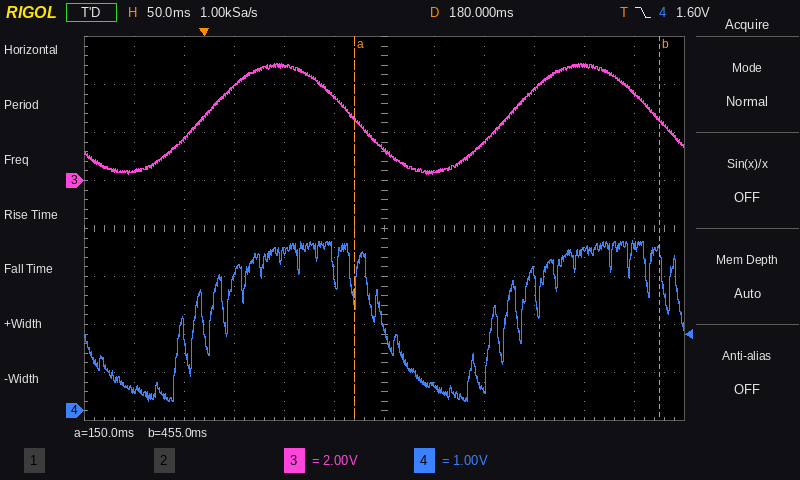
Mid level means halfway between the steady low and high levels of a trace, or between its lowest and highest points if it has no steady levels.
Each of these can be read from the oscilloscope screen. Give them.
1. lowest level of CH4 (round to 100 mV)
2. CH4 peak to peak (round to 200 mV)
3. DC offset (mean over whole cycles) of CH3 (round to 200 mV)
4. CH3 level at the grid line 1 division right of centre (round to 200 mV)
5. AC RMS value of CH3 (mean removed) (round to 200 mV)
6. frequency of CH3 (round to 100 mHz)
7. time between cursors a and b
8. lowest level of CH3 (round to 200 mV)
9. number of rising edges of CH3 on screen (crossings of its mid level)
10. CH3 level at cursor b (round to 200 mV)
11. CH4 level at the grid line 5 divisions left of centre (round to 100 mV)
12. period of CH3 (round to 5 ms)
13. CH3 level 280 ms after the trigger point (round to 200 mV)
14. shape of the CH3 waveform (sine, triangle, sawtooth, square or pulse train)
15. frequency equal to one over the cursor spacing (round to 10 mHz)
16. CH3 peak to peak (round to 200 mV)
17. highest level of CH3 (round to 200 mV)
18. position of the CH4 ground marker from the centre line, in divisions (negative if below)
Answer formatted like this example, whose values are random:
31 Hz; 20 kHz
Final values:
200 mV; 3.4 V; 2.6 V; 400 mV; 1.6 V; 3.3 Hz; 305 ms; 200 mV; 2; 2.4 V; 400 mV; 305 ms; 1.6 V; sine; 3.28 Hz; 4.6 V; 4.8 V; -3.8 div
